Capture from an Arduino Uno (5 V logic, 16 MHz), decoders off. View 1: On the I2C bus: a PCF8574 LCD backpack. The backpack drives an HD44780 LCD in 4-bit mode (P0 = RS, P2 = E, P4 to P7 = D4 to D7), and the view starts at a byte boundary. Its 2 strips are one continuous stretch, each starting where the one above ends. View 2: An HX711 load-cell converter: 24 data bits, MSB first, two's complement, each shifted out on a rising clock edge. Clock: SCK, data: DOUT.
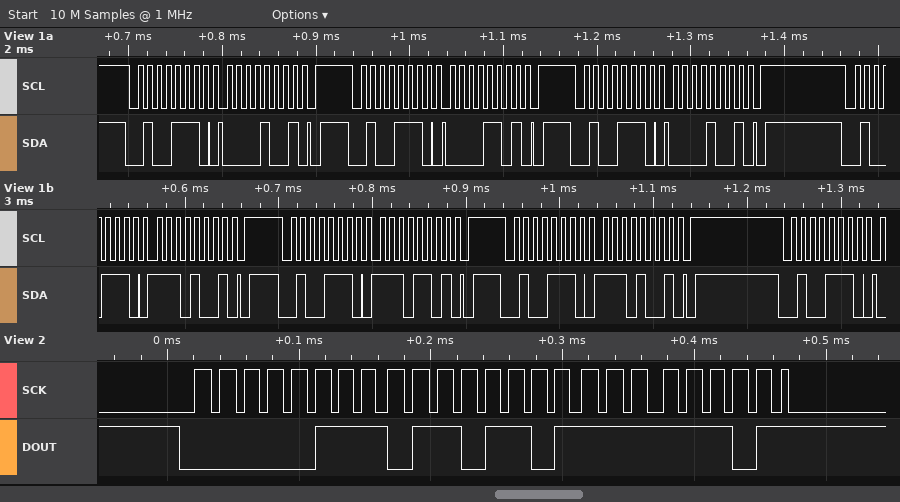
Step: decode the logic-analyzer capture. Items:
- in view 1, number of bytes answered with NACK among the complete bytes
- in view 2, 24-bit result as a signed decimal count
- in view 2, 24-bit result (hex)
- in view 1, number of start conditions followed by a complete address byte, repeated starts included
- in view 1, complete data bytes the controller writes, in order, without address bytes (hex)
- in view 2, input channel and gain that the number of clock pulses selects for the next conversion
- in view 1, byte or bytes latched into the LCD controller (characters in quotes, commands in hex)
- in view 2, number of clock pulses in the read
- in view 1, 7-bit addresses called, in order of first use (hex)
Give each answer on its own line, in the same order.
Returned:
0
486909
0x076DFD
7
09 0D 09 E9 ED E9
channel A, gain 128
data 0x0E
25
0x27
